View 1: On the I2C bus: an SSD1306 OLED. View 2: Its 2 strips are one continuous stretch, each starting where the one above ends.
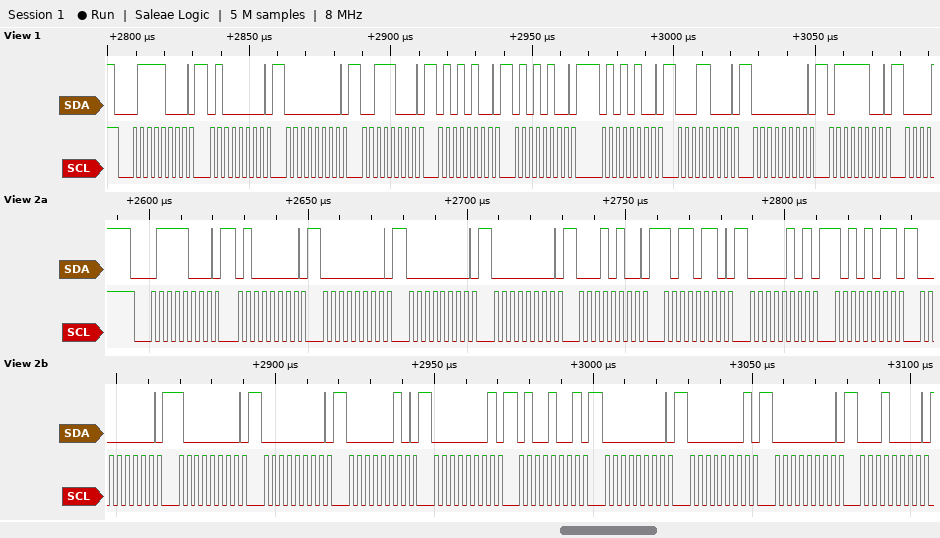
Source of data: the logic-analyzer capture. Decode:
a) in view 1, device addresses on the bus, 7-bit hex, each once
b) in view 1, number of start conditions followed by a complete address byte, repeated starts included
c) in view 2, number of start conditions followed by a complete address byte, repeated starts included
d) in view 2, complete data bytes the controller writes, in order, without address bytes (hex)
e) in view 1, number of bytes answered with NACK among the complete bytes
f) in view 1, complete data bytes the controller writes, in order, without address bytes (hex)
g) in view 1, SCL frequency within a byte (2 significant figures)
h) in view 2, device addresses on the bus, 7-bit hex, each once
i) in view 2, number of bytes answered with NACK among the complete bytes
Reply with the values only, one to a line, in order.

0x3C
1
1
40 00 00 00 14 B6 05 AB 00 80 00 02 01 49 00 01 00 10
0
40 00 38 54 54 54 18 00 7C
400 kHz
0x3C
0
